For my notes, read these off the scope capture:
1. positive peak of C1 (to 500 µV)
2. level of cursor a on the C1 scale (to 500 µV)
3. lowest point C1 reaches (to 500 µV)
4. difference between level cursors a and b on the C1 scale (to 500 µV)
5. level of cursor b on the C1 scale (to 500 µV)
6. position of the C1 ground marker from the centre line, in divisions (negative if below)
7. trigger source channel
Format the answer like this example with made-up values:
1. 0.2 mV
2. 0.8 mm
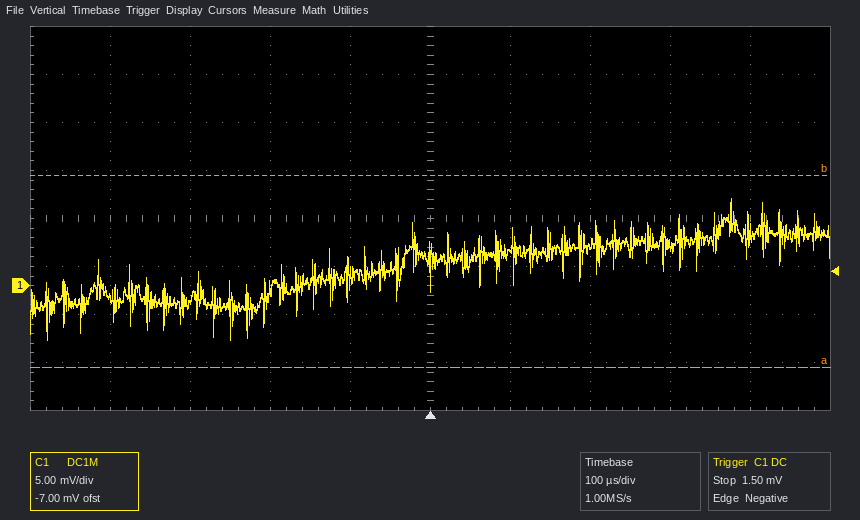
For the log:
1. 9.0 mV
2. -8.5 mV
3. -5.5 mV
4. 20.0 mV
5. 11.5 mV
6. -1.4 div
7. C1
